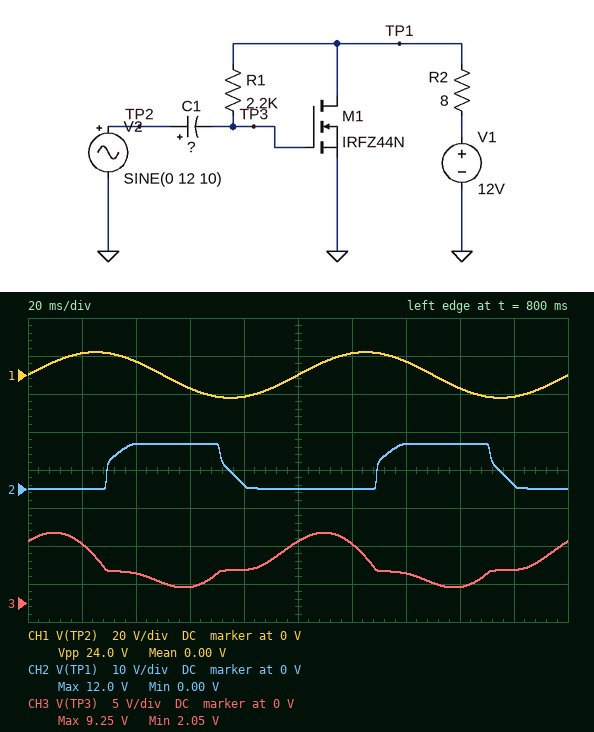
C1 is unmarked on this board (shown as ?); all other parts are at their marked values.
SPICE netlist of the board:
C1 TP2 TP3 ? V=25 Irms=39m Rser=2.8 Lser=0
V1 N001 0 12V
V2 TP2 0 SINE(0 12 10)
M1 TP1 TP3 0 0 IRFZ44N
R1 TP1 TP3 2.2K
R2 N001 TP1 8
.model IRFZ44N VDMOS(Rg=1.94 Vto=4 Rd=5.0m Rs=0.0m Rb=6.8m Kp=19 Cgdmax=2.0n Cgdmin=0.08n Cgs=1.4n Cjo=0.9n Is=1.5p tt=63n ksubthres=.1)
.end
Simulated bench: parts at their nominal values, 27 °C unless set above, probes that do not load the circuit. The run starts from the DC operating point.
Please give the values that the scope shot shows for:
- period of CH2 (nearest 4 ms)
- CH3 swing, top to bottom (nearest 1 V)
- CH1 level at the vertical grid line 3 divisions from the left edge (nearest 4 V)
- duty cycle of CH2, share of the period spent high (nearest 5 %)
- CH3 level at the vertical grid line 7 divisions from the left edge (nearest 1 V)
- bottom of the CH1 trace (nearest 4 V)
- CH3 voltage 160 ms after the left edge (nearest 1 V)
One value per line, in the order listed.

100 ms
7 V
-8 V
45 %
4 V
-12 V
2 V
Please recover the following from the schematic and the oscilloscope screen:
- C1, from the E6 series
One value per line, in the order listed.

6.8 µF
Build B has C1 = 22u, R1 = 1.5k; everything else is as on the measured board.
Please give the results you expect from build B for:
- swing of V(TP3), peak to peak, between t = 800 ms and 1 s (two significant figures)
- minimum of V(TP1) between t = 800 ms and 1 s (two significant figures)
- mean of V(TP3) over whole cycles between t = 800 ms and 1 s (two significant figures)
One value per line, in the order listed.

18 V
15 mV
5.5 V
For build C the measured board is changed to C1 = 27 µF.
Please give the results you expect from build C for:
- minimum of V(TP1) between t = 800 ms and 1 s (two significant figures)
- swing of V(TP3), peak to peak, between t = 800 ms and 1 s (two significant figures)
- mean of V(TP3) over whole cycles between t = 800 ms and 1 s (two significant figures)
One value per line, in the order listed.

14 mV
22 V
5.5 V
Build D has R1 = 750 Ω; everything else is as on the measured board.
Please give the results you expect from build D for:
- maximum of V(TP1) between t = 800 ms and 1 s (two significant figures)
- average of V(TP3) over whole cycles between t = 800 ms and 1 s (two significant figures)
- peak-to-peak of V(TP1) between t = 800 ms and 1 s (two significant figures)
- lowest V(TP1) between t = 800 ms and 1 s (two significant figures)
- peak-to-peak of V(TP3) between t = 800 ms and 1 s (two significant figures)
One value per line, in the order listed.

8.1 V
4.3 V
7.5 V
540 mV
170 mV
